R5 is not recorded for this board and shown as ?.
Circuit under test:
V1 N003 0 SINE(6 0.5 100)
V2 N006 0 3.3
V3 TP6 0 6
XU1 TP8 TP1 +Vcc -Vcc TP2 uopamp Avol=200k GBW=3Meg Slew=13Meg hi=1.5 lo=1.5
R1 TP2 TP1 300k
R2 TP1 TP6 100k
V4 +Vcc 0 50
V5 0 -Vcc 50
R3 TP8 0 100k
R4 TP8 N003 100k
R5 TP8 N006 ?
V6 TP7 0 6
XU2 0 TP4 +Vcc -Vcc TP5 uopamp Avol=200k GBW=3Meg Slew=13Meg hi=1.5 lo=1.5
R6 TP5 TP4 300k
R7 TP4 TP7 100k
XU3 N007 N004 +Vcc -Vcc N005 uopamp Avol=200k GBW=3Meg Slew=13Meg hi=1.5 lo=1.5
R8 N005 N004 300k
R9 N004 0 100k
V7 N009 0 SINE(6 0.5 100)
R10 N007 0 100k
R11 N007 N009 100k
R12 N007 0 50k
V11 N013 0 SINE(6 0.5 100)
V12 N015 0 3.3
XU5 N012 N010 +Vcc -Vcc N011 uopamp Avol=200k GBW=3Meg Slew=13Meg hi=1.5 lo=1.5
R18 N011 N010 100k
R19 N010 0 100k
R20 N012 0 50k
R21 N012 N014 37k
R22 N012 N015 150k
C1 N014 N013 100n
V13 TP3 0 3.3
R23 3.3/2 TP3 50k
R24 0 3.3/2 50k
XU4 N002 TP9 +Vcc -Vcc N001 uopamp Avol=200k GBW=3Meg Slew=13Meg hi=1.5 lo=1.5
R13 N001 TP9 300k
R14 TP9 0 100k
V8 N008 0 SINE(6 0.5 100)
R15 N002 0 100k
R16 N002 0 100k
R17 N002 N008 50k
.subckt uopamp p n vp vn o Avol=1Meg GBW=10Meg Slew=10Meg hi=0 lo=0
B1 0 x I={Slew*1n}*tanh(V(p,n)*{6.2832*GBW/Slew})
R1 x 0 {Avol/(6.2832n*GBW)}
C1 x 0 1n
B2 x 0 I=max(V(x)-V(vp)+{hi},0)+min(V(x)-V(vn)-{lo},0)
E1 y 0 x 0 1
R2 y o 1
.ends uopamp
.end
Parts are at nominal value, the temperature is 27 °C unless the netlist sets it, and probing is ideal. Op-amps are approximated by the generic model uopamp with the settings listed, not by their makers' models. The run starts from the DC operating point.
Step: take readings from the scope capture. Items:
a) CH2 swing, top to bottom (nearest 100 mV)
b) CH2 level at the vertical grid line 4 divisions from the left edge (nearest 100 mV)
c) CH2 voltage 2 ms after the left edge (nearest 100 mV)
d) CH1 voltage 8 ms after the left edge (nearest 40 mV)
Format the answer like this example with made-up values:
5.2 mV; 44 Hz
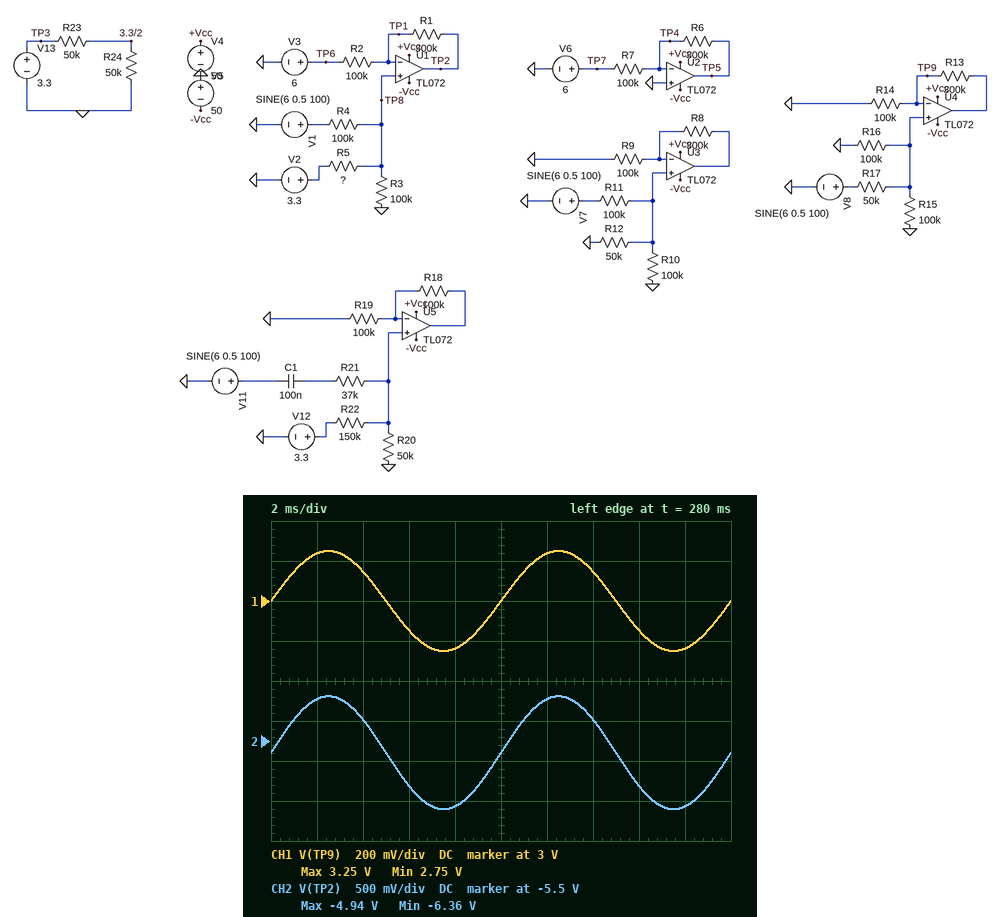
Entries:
1.4 V; -6.3 V; -5.0 V; 2.76 V
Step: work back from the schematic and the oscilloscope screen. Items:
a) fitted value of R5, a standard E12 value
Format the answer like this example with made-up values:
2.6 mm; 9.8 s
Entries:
120 kΩ
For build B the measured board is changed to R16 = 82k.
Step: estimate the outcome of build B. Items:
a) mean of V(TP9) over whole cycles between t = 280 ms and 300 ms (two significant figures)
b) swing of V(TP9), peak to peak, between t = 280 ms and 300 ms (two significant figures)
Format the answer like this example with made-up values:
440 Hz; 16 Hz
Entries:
2.8 V; 470 mV
